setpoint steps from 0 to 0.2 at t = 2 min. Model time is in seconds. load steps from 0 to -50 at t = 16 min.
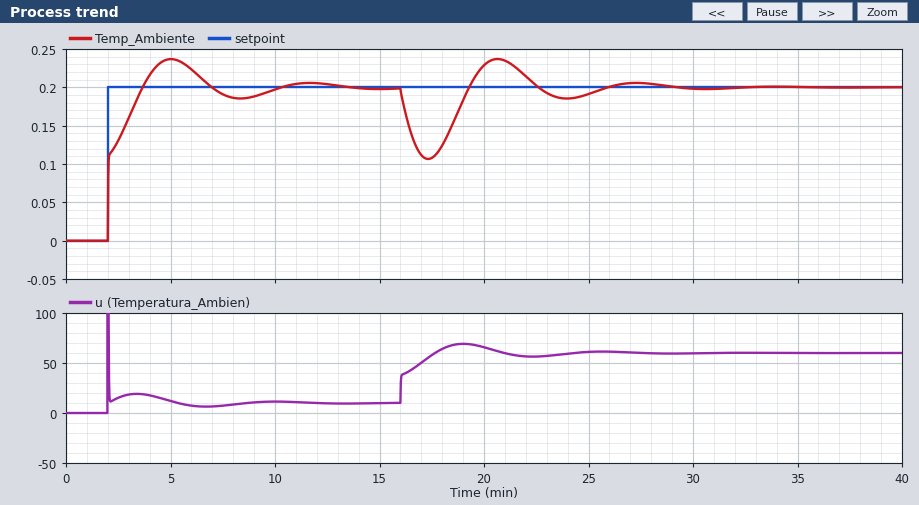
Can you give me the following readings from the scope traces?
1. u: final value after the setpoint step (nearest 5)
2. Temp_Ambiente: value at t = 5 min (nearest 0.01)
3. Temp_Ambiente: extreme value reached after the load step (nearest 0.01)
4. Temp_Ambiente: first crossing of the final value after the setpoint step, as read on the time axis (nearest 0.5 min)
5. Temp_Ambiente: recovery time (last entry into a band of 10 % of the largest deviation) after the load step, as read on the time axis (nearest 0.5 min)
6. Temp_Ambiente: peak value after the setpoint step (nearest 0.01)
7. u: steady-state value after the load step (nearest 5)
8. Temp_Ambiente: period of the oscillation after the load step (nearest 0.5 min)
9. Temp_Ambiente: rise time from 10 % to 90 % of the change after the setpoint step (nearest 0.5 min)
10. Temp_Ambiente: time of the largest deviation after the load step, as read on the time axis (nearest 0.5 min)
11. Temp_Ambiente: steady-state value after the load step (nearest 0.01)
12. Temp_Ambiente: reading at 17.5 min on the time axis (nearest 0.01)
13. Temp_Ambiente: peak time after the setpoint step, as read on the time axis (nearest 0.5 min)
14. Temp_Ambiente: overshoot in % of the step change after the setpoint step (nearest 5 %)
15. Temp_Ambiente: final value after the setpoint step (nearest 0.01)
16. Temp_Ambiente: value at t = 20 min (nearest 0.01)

10
0.24
0.11
3.5 min
25.0 min
0.24
60
6.5 min
1.5 min
17.5 min
0.20
0.11
5.0 min
20 %
0.20
0.23
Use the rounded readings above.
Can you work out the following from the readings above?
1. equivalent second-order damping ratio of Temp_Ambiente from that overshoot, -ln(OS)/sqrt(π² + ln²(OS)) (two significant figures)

0.46
